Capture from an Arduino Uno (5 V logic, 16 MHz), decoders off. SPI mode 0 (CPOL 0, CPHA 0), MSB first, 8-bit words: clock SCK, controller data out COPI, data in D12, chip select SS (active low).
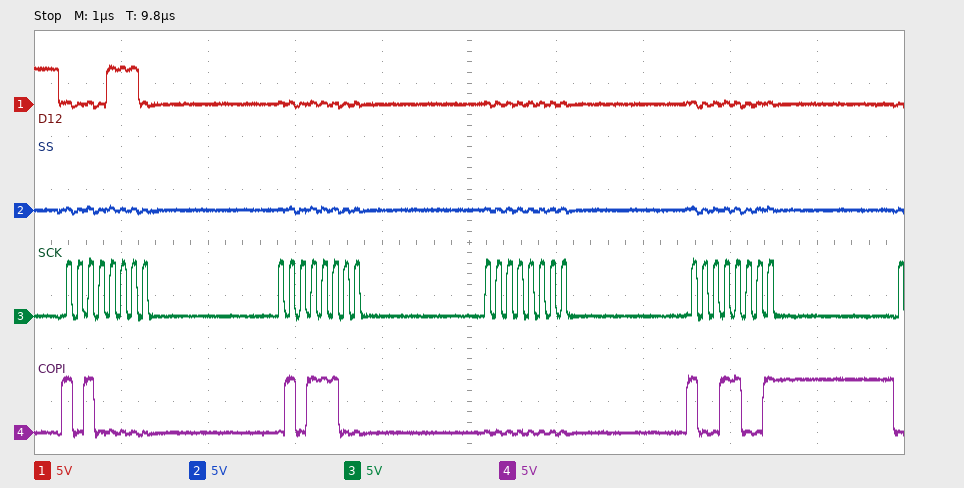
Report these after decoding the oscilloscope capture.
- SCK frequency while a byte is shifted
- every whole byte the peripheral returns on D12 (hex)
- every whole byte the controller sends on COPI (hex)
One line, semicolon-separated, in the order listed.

8 MHz; 0E 00 00 00; A0 5C 00 99
